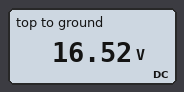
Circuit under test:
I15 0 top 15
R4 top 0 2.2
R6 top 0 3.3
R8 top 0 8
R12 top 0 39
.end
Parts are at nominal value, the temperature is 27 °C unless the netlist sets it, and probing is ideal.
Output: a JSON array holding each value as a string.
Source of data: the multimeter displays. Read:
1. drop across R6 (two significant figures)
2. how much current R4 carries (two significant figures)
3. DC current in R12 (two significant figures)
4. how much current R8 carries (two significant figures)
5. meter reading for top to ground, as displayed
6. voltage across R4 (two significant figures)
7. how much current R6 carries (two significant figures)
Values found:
["17 V", "7.5 A", "420 mA", "2.1 A", "16.52 V", "17 V", "5.0 A"]
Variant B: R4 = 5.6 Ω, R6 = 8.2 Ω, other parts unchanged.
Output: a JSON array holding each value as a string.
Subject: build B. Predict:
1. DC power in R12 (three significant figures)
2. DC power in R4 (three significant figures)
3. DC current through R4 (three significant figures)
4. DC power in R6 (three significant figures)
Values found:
["28.3 W", "197 W", "5.94 A", "135 W"]
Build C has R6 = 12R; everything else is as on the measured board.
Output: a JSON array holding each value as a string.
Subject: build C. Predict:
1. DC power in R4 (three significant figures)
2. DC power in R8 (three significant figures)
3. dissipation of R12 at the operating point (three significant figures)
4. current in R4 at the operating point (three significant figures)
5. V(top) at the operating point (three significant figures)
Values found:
["216 W", "59.3 W", "12.2 W", "9.90 A", "21.8 V"]
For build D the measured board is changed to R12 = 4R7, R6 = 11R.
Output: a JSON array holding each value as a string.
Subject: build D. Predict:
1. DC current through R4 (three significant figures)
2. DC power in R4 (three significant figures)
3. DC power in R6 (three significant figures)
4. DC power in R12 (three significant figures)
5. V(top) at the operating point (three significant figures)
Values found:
["7.72 A", "131 W", "26.2 W", "61.4 W", "17.0 V"]
